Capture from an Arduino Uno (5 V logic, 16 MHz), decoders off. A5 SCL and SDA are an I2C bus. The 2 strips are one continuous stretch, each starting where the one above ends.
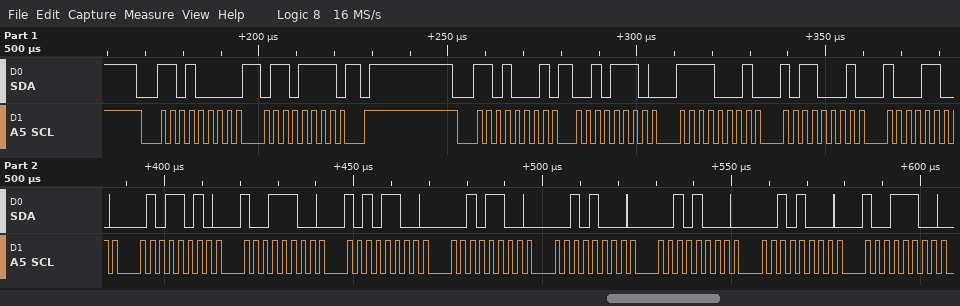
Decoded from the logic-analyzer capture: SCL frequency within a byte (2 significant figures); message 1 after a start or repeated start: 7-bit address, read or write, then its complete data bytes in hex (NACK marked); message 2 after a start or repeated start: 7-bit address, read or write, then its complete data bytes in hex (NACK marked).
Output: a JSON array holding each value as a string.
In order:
["400 kHz", "0x68 write: 6F", "0x68 read: 2E F1 B1 8C 5A 9C AC 2C 28 28 28 9C"]
